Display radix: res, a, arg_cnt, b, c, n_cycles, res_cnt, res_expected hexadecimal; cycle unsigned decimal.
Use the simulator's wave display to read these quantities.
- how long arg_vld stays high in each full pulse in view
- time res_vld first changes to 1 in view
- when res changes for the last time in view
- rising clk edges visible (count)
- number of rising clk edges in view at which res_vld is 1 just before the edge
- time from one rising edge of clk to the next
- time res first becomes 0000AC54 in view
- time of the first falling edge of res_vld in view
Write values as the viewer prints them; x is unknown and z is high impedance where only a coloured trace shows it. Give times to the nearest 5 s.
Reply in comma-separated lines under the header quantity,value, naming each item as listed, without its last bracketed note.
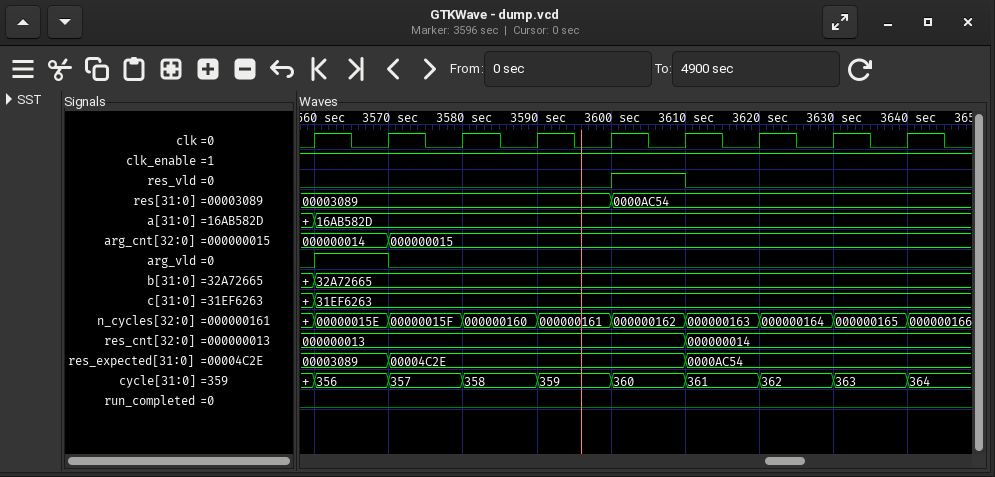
quantity,value
how long arg_vld stays high in each full pulse in view,10 s
time res_vld first changes to 1 in view,3600 s
when res changes for the last time in view,3600 s
rising clk edges visible,9
number of rising clk edges in view at which res_vld is 1 just before the edge,1
time from one rising edge of clk to the next,10 s
time res first becomes 0000AC54 in view,3600 s
time of the first falling edge of res_vld in view,3610 s
